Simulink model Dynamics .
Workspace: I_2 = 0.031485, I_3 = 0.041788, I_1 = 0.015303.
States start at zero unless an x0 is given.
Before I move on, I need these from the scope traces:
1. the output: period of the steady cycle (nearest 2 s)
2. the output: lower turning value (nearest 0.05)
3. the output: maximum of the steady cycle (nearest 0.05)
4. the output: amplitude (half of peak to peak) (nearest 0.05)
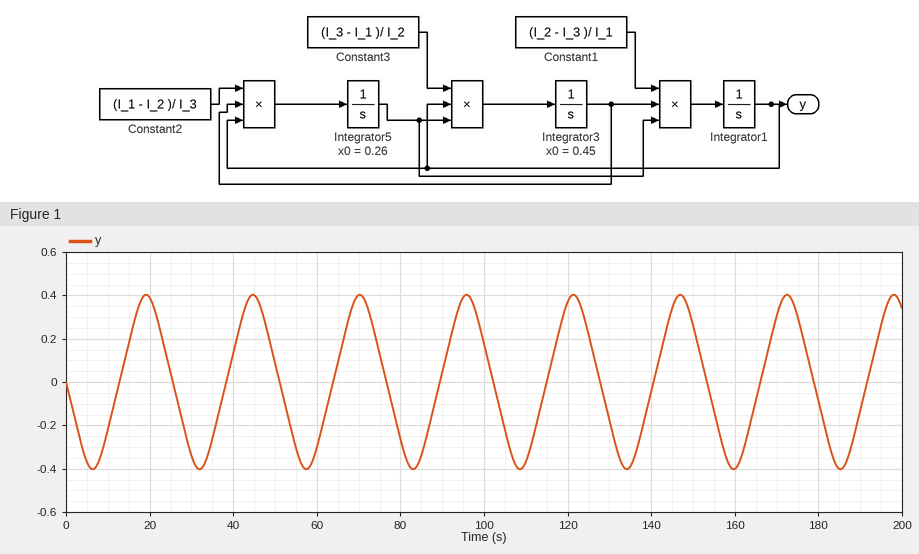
26 s
-0.40
0.40
0.40
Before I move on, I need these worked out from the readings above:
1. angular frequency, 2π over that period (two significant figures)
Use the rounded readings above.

0.24 rad/s
